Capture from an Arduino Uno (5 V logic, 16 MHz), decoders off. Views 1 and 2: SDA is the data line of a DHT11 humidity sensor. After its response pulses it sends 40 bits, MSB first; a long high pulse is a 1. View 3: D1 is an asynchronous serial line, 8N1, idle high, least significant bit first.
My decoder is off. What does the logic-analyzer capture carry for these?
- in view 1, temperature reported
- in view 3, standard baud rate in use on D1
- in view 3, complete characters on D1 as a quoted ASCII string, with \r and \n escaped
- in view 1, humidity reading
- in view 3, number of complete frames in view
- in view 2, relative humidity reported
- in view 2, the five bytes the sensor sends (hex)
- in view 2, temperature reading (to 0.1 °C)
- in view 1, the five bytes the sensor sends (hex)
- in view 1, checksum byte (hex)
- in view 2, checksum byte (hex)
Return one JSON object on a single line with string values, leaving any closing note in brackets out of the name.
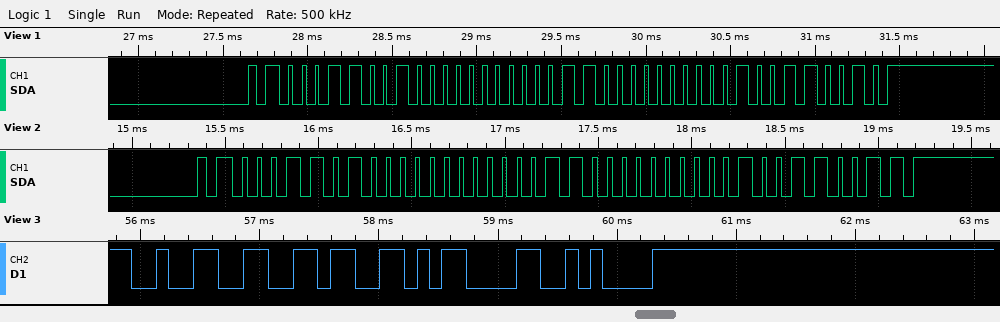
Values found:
{"in view 1, temperature reported": "24.1 °C", "in view 3, standard baud rate in use on D1": "9600 baud", "in view 3, complete characters on D1 as a quoted ASCII string, with \\r and \\n escaped": "\"26\\r\\n\"", "in view 1, humidity reading": "25 %", "in view 3, number of complete frames in view": "4", "in view 2, relative humidity reported": "26 %", "in view 2, the five bytes the sensor sends": "1A 00 18 01 33", "in view 2, temperature reading": "24.1 °C", "in view 1, the five bytes the sensor sends": "19 00 18 01 32", "in view 1, checksum byte": "0x32", "in view 2, checksum byte": "0x33"}
